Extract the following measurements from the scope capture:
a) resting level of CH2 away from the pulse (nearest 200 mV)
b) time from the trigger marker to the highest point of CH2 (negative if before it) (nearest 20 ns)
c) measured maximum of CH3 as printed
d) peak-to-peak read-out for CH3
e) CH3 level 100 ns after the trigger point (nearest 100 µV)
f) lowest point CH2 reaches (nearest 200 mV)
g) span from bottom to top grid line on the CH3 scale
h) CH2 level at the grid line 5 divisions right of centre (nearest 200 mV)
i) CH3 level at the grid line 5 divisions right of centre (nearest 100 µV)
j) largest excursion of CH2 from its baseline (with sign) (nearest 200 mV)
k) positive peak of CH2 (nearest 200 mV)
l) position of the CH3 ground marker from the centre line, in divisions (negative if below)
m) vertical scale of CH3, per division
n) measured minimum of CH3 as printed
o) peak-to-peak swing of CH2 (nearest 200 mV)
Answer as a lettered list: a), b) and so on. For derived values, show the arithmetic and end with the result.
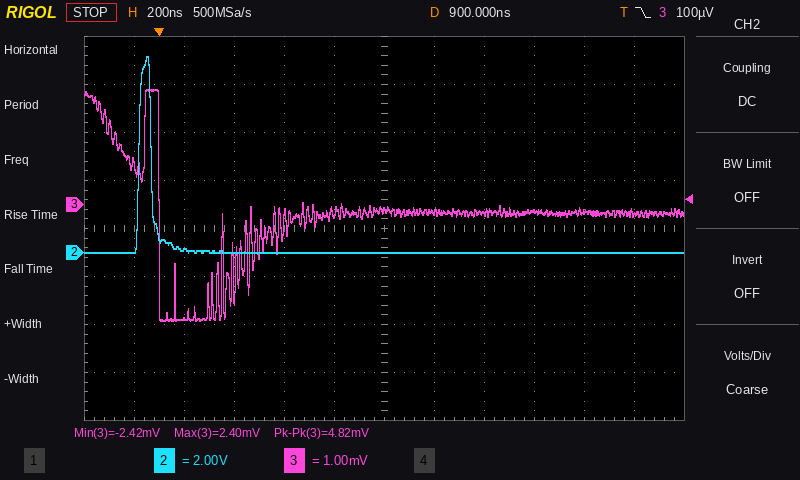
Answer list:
a) 0.0 V
b) -40 ns
c) 2.40 mV
d) 4.82 mV
e) -2.4 mV
f) 0.0 V
g) 8 mV
h) 0.0 V
i) -200 µV
j) 8.2 V − (0.0 V) = +8.2 V
k) 8.2 V
l) +0.5 div
m) 1 mV
n) -2.42 mV
o) 8.2 V − (0.0 V) = 8.2 V
